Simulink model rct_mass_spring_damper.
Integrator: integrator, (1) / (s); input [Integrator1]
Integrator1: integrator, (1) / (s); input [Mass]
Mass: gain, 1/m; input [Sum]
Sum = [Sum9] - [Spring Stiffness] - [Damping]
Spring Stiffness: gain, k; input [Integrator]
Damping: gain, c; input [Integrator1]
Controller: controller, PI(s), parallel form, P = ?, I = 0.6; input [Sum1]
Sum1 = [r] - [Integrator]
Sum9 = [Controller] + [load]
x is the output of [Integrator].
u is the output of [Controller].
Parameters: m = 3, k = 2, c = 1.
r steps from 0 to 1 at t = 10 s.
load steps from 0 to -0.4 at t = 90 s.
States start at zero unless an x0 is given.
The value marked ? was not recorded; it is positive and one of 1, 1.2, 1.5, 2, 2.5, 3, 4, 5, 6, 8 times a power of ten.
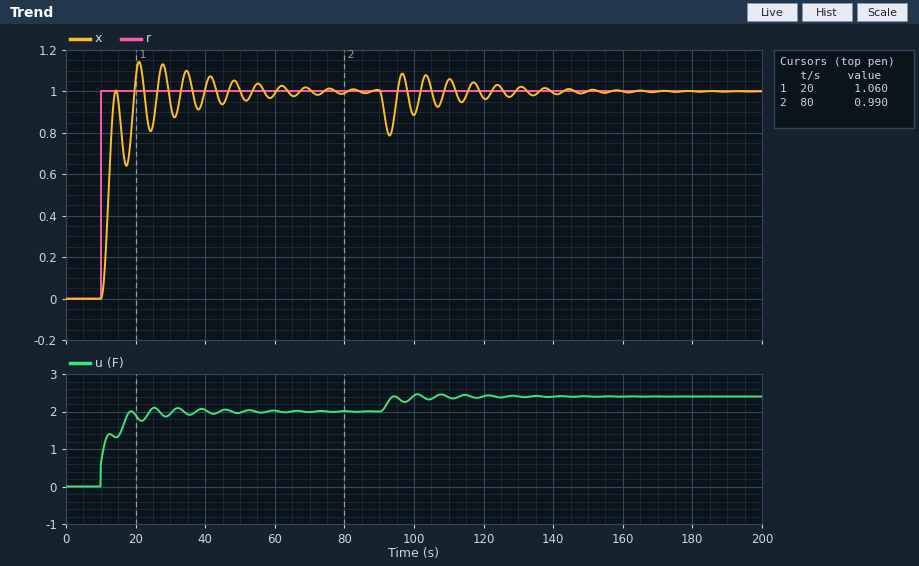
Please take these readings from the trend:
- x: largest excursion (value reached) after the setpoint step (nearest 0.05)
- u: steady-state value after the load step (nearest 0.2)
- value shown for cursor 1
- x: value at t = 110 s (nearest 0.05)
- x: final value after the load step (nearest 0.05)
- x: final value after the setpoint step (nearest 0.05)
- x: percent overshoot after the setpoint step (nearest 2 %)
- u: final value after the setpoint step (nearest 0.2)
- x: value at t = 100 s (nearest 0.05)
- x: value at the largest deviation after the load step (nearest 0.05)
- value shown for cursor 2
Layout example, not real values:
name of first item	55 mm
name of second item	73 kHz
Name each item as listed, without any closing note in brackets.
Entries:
x: largest excursion (value reached) after the setpoint step	1.15
u: steady-state value after the load step	2.4
value shown for cursor 1	1.060
x: value at t = 110 s	1.05
x: final value after the load step	1.00
x: final value after the setpoint step	1.00
x: percent overshoot after the setpoint step	14 %
u: final value after the setpoint step	2.0
x: value at t = 100 s	0.90
x: value at the largest deviation after the load step	0.80
value shown for cursor 2	0.990
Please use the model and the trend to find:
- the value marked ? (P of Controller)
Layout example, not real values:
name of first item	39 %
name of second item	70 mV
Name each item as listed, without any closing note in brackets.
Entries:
the value marked ?	0.6
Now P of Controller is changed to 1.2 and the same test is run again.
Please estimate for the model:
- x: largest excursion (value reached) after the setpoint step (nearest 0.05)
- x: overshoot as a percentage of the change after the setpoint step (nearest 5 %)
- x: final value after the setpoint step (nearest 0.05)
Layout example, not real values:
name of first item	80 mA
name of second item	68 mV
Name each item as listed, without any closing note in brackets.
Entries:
x: largest excursion (value reached) after the setpoint step	1.10
x: overshoot as a percentage of the change after the setpoint step	10 %
x: final value after the setpoint step	1.00
